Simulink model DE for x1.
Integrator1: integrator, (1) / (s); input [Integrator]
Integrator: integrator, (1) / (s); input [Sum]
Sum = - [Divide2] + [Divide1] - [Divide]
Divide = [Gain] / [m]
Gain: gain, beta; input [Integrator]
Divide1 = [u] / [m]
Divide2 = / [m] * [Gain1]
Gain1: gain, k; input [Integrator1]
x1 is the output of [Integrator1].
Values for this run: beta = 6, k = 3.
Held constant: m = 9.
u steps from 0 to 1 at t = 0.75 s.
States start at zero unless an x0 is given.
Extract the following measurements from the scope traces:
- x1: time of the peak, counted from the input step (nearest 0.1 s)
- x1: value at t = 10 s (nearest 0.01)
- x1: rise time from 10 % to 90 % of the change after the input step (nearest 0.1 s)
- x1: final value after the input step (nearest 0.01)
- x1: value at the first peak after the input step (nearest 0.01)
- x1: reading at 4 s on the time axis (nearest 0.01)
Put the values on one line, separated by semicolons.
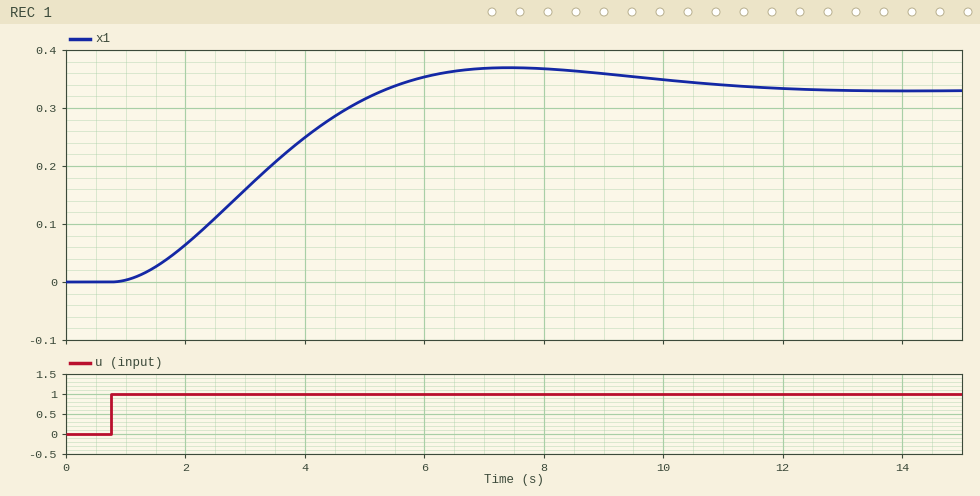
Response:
6.7 s; 0.35; 3.1 s; 0.33; 0.37; 0.25
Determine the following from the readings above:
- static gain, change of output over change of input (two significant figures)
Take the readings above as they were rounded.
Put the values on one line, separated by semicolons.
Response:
0.33
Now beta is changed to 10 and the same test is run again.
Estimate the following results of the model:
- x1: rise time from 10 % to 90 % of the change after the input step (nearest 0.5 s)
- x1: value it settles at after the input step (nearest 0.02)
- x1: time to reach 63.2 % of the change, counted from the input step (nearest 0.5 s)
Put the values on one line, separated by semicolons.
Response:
5.5 s; 0.34; 3.5 s
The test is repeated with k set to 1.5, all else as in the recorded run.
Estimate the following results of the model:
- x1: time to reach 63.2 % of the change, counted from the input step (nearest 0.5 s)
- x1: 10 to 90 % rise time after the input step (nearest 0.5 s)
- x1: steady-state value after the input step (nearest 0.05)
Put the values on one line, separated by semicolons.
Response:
4.5 s; 6.0 s; 0.65
